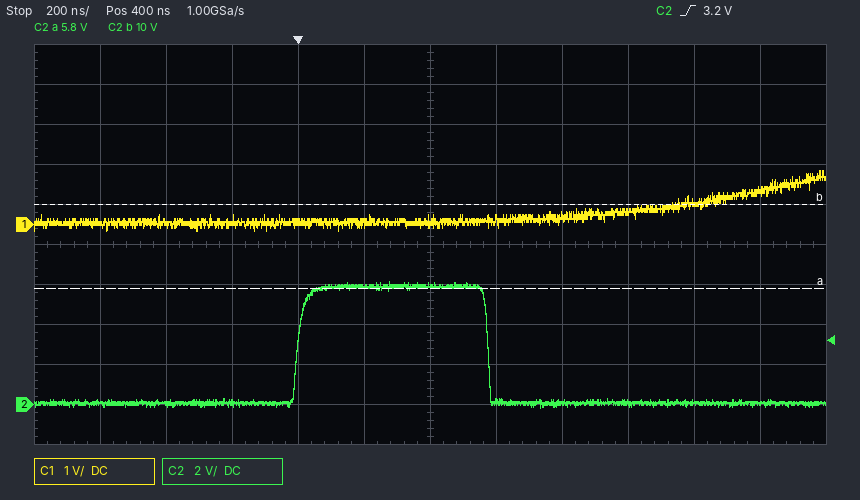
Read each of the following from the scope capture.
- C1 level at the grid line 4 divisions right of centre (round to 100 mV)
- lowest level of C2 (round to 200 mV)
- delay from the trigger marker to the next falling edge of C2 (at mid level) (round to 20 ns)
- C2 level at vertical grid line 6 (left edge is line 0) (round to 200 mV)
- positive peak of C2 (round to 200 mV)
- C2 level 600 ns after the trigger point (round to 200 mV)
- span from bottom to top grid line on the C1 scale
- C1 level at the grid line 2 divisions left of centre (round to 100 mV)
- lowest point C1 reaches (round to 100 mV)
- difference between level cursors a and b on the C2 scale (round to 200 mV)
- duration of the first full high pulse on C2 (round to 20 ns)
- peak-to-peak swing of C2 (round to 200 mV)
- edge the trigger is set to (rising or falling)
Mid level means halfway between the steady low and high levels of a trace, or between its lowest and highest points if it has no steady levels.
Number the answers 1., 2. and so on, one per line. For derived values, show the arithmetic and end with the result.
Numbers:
1. 600 mV
2. -200 mV
3. 580 ns
4. 6.0 V
5. 6.2 V
6. 200 mV
7. 10 V
8. 100 mV
9. -200 mV
10. 4.2 V
11. 580 ns
12. 6.2 V − (-200 mV) = 6.4 V
13. rising
